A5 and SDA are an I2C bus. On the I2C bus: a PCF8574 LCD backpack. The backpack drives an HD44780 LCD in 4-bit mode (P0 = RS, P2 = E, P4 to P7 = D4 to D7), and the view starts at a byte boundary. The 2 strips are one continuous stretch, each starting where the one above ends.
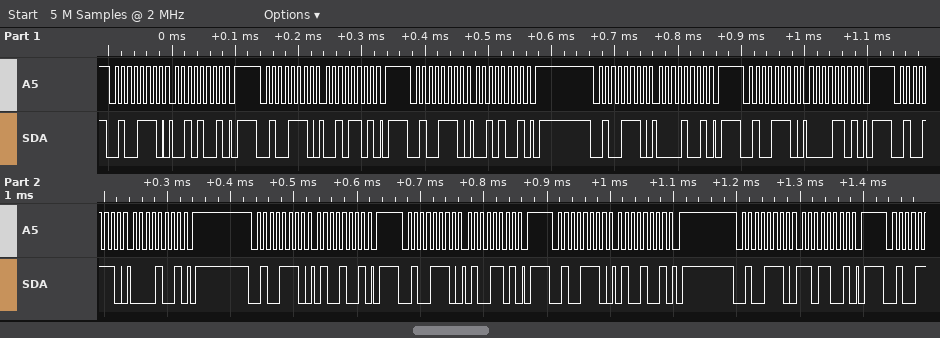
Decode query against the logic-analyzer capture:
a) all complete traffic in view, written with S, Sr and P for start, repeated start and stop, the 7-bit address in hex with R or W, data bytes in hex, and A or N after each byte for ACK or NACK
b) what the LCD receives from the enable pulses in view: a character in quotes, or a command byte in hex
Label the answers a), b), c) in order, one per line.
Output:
a) S 27W A 29 A P S 27W A 2D A P S 27W A 29 A P S 27W A 09 A P S 27W A 0D A P S 27W A 09 A P S 27W A 49 A P S 27W A 4D A P S 27W A 49 A P S 27W A D9 A P
b) ' '
